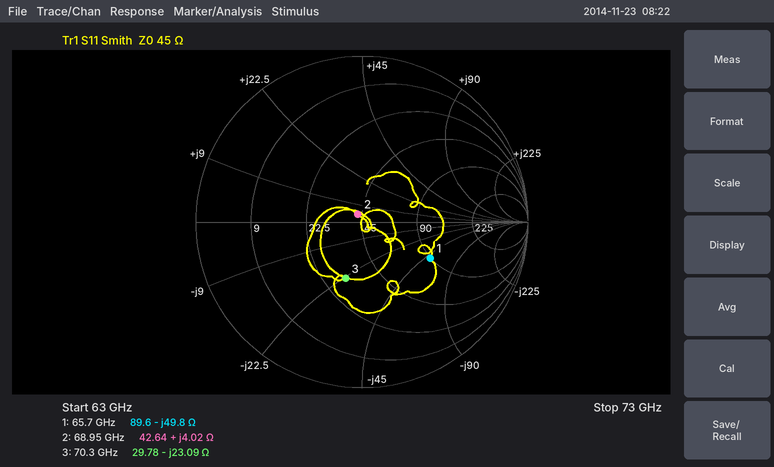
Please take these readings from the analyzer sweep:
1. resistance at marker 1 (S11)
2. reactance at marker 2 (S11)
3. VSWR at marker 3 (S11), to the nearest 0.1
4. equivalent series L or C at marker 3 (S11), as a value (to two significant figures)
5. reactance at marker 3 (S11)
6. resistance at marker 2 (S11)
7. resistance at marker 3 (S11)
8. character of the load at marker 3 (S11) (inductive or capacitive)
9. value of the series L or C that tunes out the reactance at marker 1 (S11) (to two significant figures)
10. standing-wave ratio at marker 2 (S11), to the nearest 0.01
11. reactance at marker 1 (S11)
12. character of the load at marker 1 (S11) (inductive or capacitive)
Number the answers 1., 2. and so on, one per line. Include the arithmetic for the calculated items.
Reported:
1. 89.6 Ω
2. +4.02 Ω
3. 2.1
4. C = 1/(2π × 70.3 GHz × 23.09 Ω) ≈ 98 fF
5. -23.09 Ω
6. 42.64 Ω
7. 29.78 Ω
8. capacitive
9. L = 49.8 Ω/(2π × 65.7 GHz) ≈ 121 pH, so 120 pH to two significant figures
10. 1.11
11. -49.8 Ω
12. capacitive
